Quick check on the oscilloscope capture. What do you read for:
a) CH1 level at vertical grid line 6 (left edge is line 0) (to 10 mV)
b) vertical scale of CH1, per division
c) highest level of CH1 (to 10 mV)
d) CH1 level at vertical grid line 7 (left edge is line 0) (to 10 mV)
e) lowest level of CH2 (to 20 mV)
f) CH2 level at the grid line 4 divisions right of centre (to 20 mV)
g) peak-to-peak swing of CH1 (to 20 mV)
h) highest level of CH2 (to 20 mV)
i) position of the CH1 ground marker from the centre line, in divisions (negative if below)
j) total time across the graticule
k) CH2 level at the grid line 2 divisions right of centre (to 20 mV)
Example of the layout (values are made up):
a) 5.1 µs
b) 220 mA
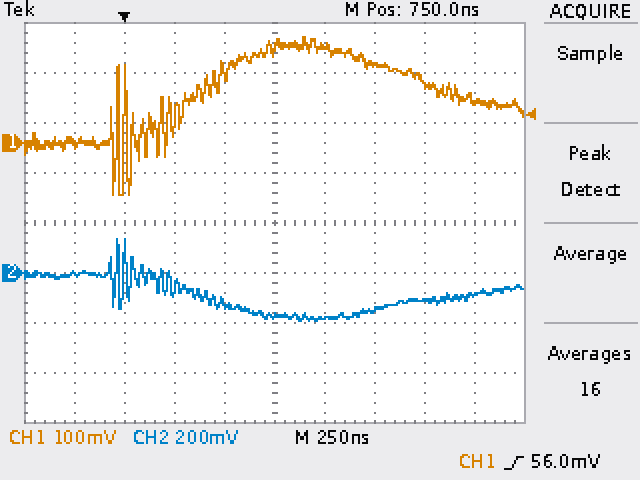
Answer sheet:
a) 190 mV
b) 100 mV
c) 210 mV
d) 160 mV
e) -200 mV
f) -80 mV
g) 320 mV
h) 140 mV
i) +1.6 div
j) 2.5 µs
k) -140 mV
